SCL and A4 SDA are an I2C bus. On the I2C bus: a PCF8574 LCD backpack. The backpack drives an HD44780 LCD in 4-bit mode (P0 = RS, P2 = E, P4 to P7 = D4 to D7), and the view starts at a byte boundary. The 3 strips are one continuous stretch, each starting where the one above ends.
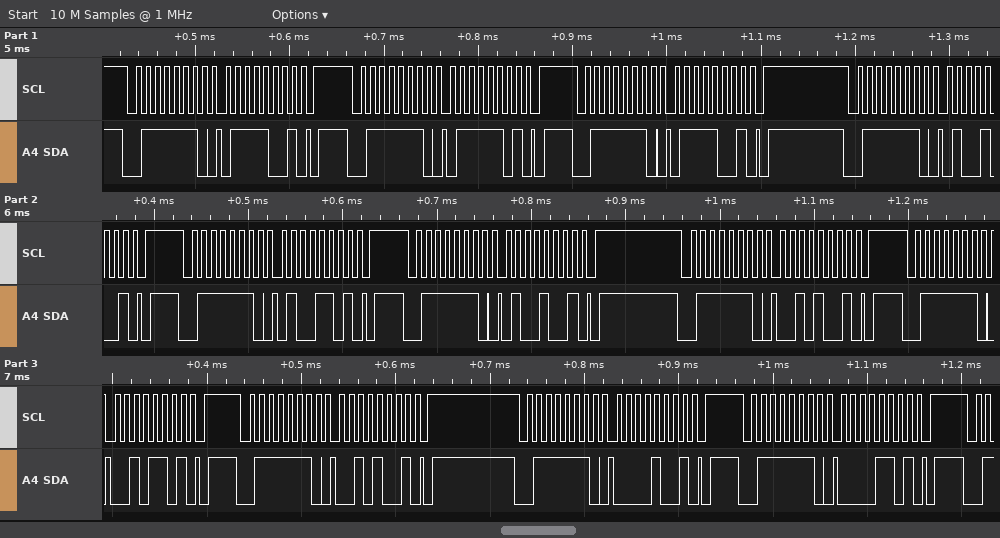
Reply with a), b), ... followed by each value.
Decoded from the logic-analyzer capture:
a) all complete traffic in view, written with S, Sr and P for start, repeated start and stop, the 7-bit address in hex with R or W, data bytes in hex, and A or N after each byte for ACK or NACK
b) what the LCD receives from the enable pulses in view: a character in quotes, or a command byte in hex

a) S 3FW A 79 A P S 3FW A 7D A P S 3FW A 79 A P S 3FW A 49 A P S 3FW A 4D A P S 3FW A 49 A P S 3FW A 29 A P S 3FW A 2D A P S 3FW A 29 A P S 3FW A 09 A P S 3FW A 0D A P
b) 't'
